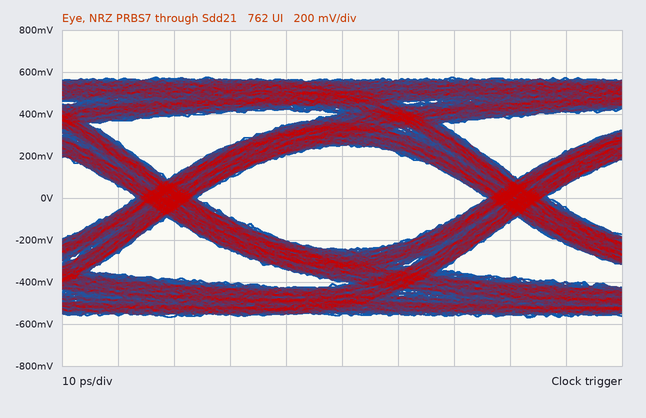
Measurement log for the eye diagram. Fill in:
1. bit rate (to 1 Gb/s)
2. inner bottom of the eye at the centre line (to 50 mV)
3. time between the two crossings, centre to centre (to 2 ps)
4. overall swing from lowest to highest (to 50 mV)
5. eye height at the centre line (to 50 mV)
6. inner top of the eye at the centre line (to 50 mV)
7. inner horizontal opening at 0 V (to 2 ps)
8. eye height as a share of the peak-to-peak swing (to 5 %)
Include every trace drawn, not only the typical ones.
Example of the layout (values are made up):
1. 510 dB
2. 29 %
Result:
1. 16 Gb/s
2. -250 mV
3. 62 ps
4. 1.15 V
5. 500 mV
6. 250 mV
7. 52 ps
8. 45 %
